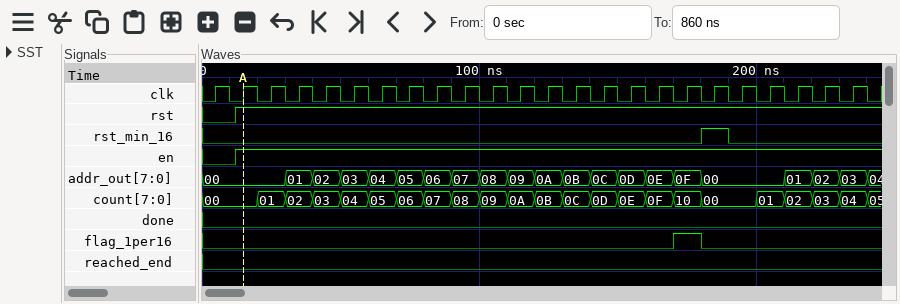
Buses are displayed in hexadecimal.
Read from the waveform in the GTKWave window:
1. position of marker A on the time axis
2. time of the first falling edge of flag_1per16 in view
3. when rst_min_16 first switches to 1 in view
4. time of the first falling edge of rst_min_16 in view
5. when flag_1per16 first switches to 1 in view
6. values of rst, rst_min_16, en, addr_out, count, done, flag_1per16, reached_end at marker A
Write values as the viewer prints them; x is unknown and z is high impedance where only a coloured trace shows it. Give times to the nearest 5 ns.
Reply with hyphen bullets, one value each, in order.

- 15 ns
- 180 ns
- 180 ns
- 190 ns
- 170 ns
- rst=1, rst_min_16=0, en=1, addr_out=00, count=00, done=0, flag_1per16=0, reached_end=0
